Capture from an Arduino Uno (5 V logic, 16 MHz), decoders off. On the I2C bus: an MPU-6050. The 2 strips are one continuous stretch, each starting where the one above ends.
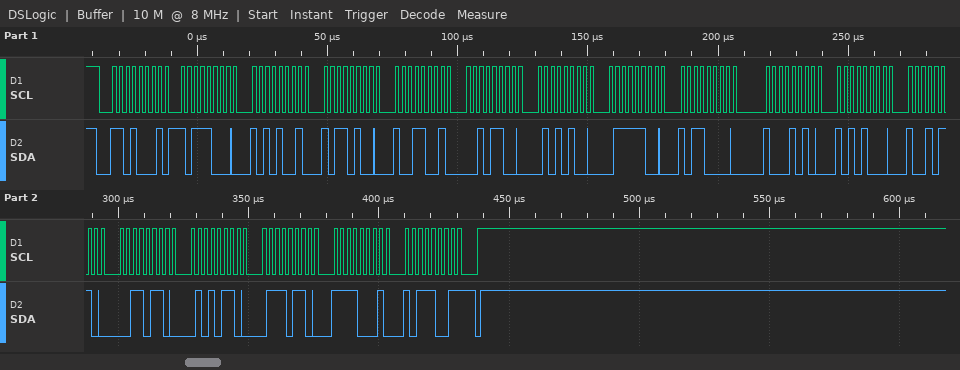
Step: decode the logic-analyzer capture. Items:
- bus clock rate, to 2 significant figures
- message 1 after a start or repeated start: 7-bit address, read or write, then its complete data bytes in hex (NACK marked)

400 kHz
0x68 read: B8 A9 B4 99 2C 54 7C B0 8A A8 96 36 56 76 F1 B9 NACK
